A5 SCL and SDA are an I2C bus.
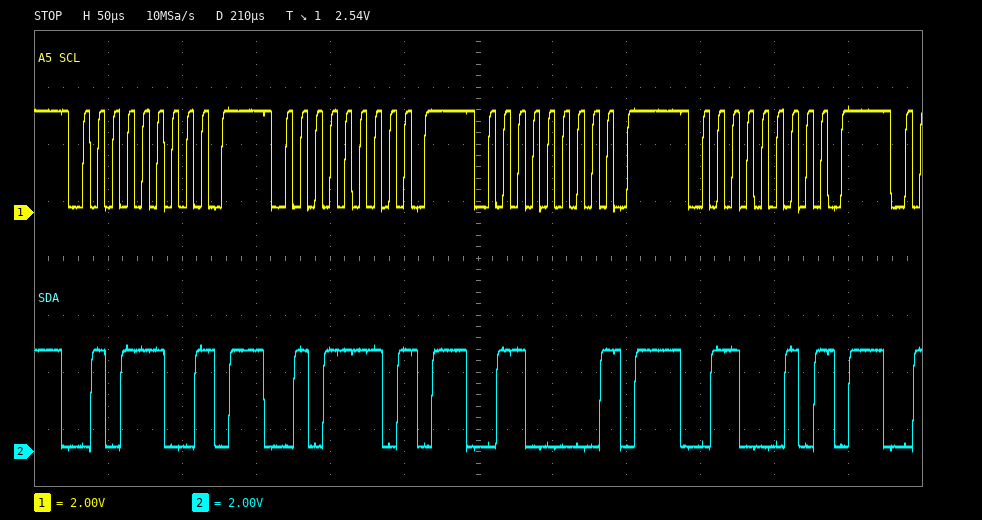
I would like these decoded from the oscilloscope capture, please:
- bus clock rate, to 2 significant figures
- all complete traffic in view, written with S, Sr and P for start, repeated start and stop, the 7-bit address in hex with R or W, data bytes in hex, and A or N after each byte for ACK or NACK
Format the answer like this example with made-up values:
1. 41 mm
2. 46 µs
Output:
1. 100 kHz
2. S 2EW N P S 2FW N P S 30W N P S 31W N P
